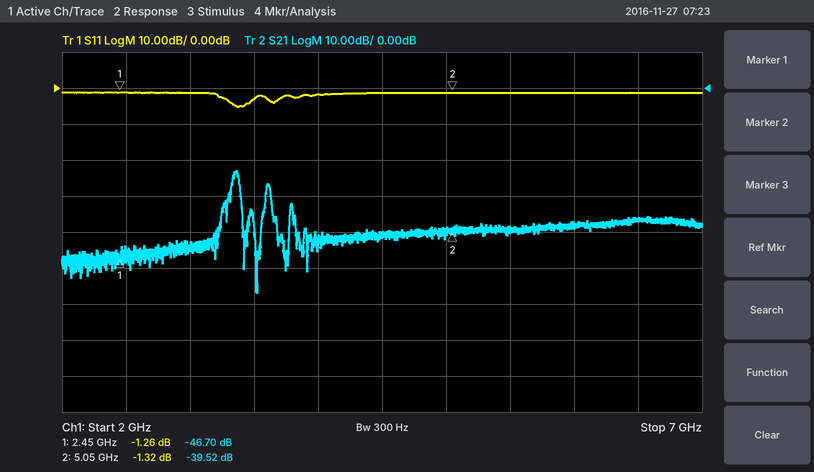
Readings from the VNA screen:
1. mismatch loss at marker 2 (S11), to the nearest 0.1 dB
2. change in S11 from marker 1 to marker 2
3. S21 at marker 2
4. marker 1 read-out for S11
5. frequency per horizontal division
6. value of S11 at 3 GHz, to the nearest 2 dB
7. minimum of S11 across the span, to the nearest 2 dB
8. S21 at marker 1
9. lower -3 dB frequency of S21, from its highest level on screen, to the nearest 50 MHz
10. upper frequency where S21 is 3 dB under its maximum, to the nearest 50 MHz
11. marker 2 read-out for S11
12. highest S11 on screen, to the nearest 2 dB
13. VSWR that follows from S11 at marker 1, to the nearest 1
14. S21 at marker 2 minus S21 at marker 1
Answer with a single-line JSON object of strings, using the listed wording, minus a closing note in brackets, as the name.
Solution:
{"mismatch loss at marker 2 (S11), to the nearest 0.1 dB": "5.8 dB", "change in S11 from marker 1 to marker 2": "-0.06 dB", "S21 at marker 2": "-39.52 dB", "marker 1 read-out for S11": "-1.26 dB", "frequency per horizontal division": "500 MHz", "value of S11 at 3 GHz, to the nearest 2 dB": "-2 dB", "minimum of S11 across the span, to the nearest 2 dB": "-6 dB", "S21 at marker 1": "-46.70 dB", "lower -3 dB frequency of S21, from its highest level on screen, to the nearest 50 MHz": "3.35 GHz", "upper frequency where S21 is 3 dB under its maximum, to the nearest 50 MHz": "3.40 GHz", "marker 2 read-out for S11": "-1.32 dB", "highest S11 on screen, to the nearest 2 dB": "-2 dB", "VSWR that follows from S11 at marker 1, to the nearest 1": "14", "S21 at marker 2 minus S21 at marker 1": "7.18 dB"}
